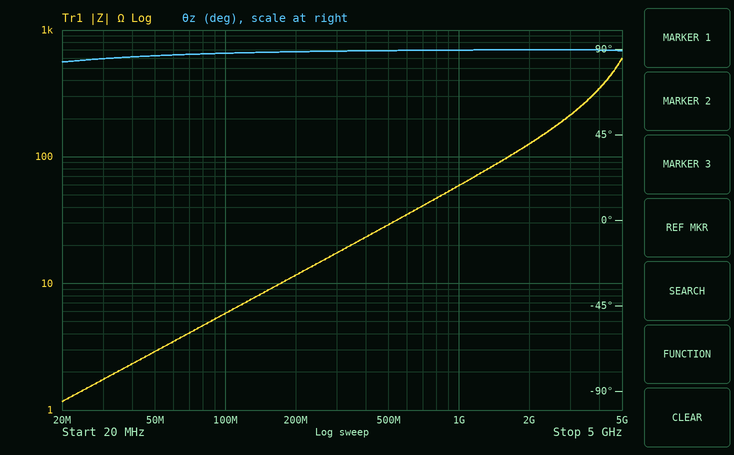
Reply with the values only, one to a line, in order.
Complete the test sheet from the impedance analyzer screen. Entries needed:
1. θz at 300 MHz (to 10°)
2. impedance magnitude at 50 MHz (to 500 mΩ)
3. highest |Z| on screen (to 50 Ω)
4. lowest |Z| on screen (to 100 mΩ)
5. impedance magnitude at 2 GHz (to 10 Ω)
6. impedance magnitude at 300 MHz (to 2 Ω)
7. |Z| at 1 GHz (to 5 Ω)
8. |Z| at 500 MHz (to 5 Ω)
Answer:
90°
3.0 Ω
600 Ω
1.2 Ω
130 Ω
18 Ω
60 Ω
30 Ω
